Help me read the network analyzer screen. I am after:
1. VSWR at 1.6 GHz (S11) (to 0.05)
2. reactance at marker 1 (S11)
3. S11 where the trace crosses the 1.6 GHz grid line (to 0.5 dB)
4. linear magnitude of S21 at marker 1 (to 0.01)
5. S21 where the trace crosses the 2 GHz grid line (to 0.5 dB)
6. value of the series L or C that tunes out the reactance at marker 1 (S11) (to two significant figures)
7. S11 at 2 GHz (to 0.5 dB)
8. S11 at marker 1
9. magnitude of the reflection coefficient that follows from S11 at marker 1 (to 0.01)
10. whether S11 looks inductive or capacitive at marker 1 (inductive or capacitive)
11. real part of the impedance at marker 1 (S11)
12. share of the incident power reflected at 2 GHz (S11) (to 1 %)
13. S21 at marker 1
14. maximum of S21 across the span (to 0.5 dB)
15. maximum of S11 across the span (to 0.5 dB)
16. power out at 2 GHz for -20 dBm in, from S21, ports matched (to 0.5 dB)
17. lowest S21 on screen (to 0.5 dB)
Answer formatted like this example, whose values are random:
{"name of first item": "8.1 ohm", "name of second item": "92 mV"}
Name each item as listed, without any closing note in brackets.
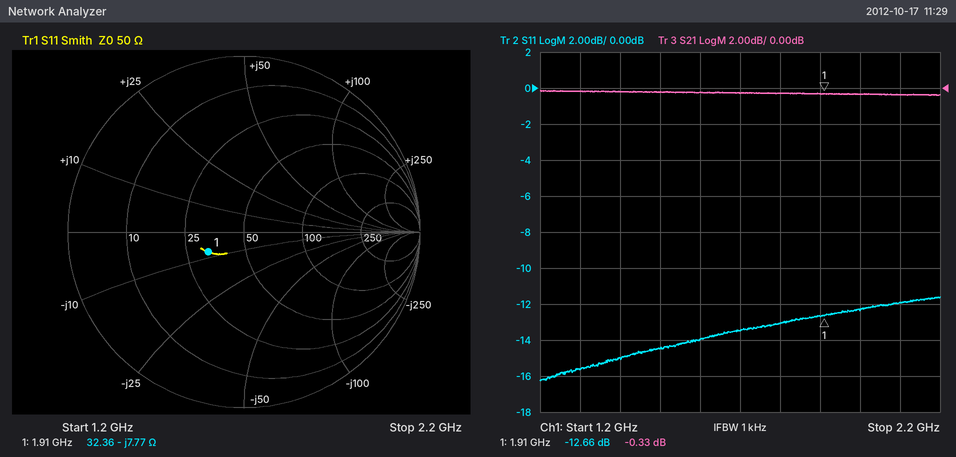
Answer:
{"VSWR at 1.6 GHz (S11)": "1.50", "reactance at marker 1": "-7.77 Ω", "S11 where the trace crosses the 1.6 GHz grid line": "-14.0 dB", "linear magnitude of S21 at marker 1": "0.96", "S21 where the trace crosses the 2 GHz grid line": "-0.5 dB", "value of the series L or C that tunes out the reactance at marker 1 (S11)": "650 pH", "S11 at 2 GHz": "-12.5 dB", "S11 at marker 1": "-12.66 dB", "magnitude of the reflection coefficient that follows from S11 at marker 1": "0.23", "whether S11 looks inductive or capacitive at marker 1": "capacitive", "real part of the impedance at marker 1": "32.36 Ω", "share of the incident power reflected at 2 GHz (S11)": "6 %", "S21 at marker 1": "-0.33 dB", "maximum of S21 across the span": "0.0 dB", "maximum of S11 across the span": "-11.5 dB", "power out at 2 GHz for -20 dBm in, from S21, ports matched": "-20.5 dBm", "lowest S21 on screen": "-0.5 dB"}
